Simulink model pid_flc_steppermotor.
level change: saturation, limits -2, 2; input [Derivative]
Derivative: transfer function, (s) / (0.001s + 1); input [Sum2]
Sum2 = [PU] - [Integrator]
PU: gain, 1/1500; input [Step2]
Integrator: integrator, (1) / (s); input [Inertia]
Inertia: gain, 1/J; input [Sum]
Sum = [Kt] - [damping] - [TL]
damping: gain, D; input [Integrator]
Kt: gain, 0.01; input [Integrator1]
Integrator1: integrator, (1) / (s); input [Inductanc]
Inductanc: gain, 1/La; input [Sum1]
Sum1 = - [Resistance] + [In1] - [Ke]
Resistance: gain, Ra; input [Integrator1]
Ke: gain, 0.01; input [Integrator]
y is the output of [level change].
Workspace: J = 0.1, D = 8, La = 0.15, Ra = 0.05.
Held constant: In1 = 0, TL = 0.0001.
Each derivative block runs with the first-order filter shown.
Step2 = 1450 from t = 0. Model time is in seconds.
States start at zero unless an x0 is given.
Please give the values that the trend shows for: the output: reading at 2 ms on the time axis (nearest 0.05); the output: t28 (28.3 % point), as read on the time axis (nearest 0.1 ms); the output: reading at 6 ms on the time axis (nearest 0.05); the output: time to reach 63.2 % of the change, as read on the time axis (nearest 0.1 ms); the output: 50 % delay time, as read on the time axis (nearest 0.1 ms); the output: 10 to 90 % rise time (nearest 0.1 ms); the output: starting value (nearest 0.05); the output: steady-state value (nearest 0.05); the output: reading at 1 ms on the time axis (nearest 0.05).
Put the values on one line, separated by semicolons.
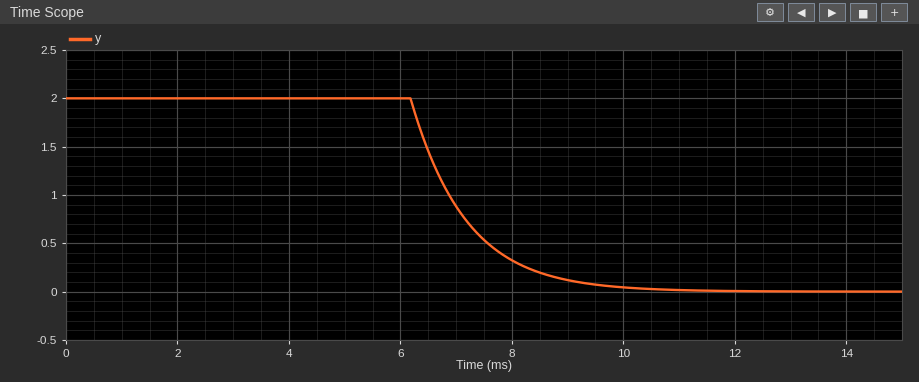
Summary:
2.00; 6.5 ms; 2.00; 7.2 ms; 6.9 ms; 2.2 ms; 2.00; 0.00; 2.00
